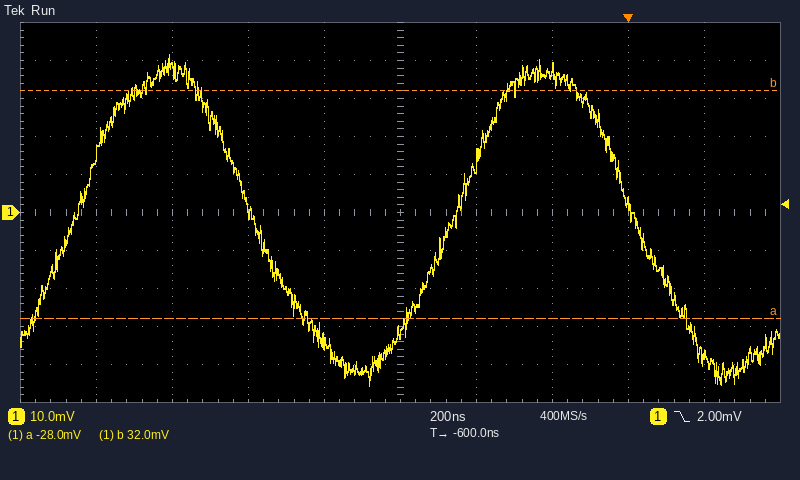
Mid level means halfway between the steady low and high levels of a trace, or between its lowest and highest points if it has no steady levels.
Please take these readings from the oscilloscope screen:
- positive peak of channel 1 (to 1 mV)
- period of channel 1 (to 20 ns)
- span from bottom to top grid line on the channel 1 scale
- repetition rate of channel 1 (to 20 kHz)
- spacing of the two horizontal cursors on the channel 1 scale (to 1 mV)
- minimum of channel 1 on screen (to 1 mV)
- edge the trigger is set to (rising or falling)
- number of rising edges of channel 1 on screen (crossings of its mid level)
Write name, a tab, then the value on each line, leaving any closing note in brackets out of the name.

positive peak of channel 1	42 mV
period of channel 1	1.00 µs
span from bottom to top grid line on the channel 1 scale	100 mV
repetition rate of channel 1	1.00 MHz
spacing of the two horizontal cursors on the channel 1 scale	60 mV
minimum of channel 1 on screen	-46 mV
edge the trigger is set to	falling
number of rising edges of channel 1 on screen	2
